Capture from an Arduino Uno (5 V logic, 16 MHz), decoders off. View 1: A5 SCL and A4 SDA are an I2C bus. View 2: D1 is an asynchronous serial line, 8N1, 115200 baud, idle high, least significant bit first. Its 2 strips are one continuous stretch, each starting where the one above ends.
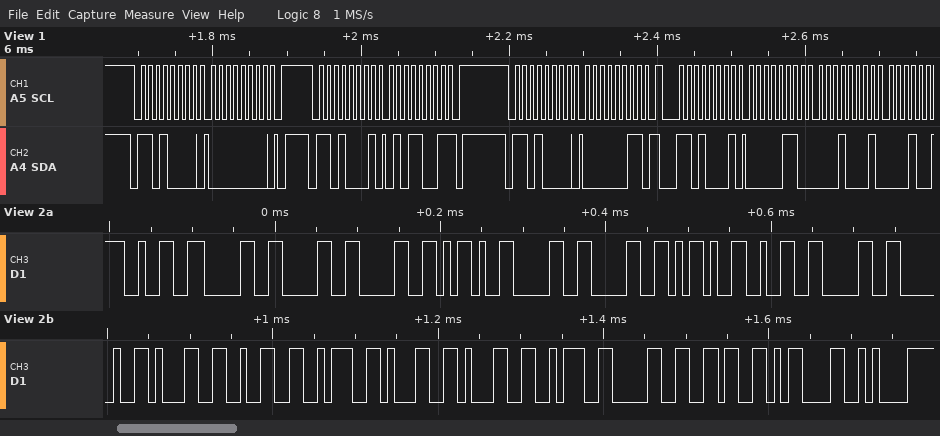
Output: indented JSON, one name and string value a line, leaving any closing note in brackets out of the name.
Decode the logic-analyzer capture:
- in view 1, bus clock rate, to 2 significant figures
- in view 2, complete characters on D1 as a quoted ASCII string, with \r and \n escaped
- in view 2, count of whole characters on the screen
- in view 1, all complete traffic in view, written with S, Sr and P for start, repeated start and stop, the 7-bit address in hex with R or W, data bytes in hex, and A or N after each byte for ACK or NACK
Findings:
{
  "in view 1, bus clock rate, to 2 significant figures": "100 kHz",
  "in view 2, complete characters on D1 as a quoted ASCII string, with \\r and \\n escaped": "\"2000-00-20 12:11:06\\r\\n\"",
  "in view 2, count of whole characters on the screen": "21",
  "in view 1, all complete traffic in view, written with S, Sr and P for start, repeated start and stop, the 7-bit address in hex with R or W, data bytes in hex, and A or N after each byte for ACK or NACK": "S 68W A 00 A P S 68R A 59 N P S 68W A 03 A Sr 68R A 06 A 11 A"
}
